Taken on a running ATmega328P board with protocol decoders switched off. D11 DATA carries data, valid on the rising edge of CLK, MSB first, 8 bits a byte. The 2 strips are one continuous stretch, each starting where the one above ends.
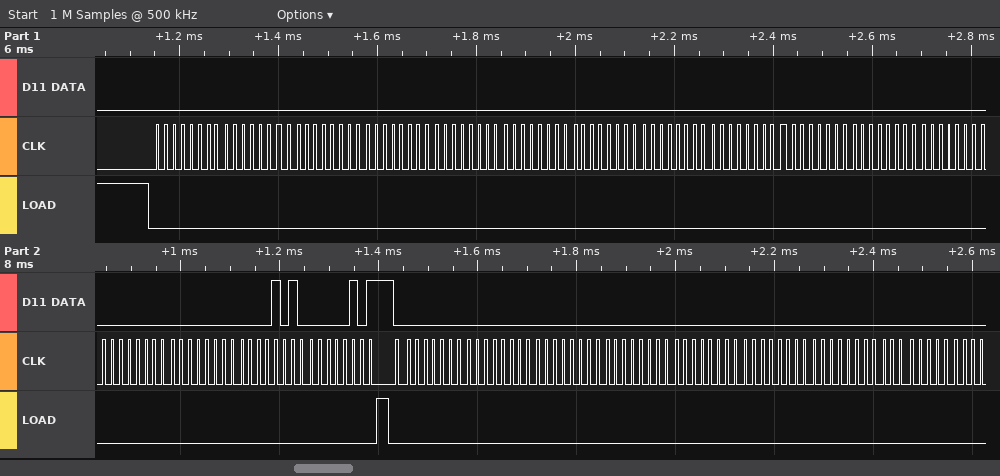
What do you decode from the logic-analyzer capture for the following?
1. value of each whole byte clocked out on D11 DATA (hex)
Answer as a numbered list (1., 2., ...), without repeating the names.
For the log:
1. 00 00 00 00 00 00 00 00 00 00 00 00 00 00 0A 05 00 00 00 00 00 00 00 00
